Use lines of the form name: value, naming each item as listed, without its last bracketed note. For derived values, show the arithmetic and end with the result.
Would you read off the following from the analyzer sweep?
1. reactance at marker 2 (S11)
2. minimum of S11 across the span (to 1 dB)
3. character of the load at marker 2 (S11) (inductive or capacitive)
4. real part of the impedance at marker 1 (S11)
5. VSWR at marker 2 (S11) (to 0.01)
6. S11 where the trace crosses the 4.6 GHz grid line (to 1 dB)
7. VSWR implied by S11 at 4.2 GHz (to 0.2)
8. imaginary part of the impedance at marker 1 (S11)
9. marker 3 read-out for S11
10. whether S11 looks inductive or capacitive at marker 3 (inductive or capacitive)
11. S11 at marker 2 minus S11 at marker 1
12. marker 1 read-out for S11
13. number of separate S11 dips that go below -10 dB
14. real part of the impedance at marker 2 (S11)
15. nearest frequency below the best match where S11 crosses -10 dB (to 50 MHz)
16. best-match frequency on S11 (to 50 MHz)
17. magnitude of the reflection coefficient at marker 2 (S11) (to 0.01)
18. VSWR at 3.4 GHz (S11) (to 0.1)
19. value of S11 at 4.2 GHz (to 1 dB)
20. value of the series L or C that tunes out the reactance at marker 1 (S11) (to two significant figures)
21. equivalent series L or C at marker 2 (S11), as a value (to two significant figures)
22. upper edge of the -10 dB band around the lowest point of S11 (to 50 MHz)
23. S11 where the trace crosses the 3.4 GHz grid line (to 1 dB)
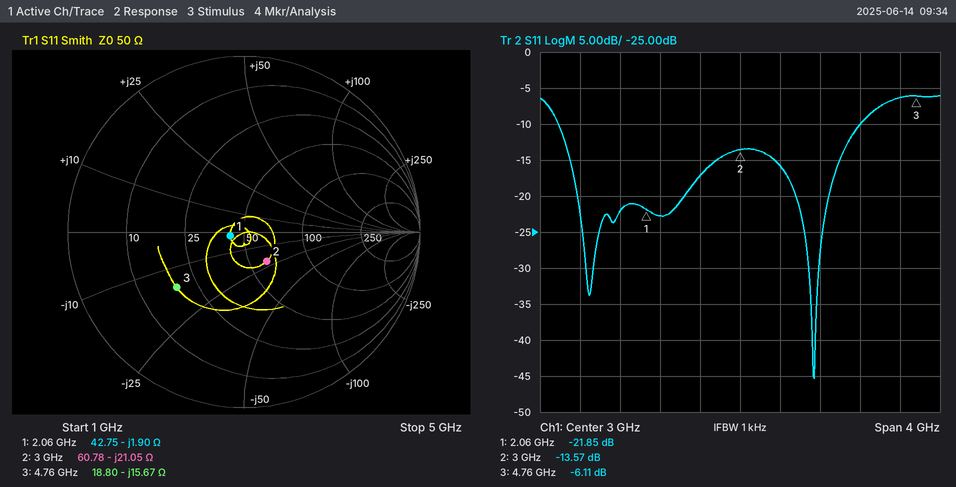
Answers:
reactance at marker 2: -21.05 Ω
minimum of S11 across the span: -45 dB
character of the load at marker 2 (S11): capacitive
real part of the impedance at marker 1: 42.75 Ω
VSWR at marker 2 (S11): (1 + 0.2097)/(1 − 0.2097) ≈ 1.53
S11 where the trace crosses the 4.6 GHz grid line: -6 dB
VSWR implied by S11 at 4.2 GHz: |Γ| = 10^(-10/20) = 0.3162; VSWR = (1 + 0.3162)/(1 − 0.3162) ≈ 1.92, so 2.0 to the nearest 0.2
imaginary part of the impedance at marker 1: -1.90 Ω
marker 3 read-out for S11: -6.11 dB
whether S11 looks inductive or capacitive at marker 3: capacitive
S11 at marker 2 minus S11 at marker 1: -13.57 − (-21.85) = 8.28 dB
marker 1 read-out for S11: -21.85 dB
number of separate S11 dips that go below -10 dB: 2
real part of the impedance at marker 2: 60.78 Ω
nearest frequency below the best match where S11 crosses -10 dB: 1.20 GHz
best-match frequency on S11: 3.75 GHz
magnitude of the reflection coefficient at marker 2 (S11): 0.21
VSWR at 3.4 GHz (S11): |Γ| = 10^(-16/20) = 0.1585; VSWR = (1 + 0.1585)/(1 − 0.1585) ≈ 1.4
value of S11 at 4.2 GHz: -10 dB
value of the series L or C that tunes out the reactance at marker 1 (S11): L = 1.9 Ω/(2π × 2.06 GHz) ≈ 147 pH, so 150 pH to two significant figures
equivalent series L or C at marker 2 (S11), as a value: C = 1/(2π × 3 GHz × 21.05 Ω) ≈ 2.5 pF
upper edge of the -10 dB band around the lowest point of S11: 4.20 GHz
S11 where the trace crosses the 3.4 GHz grid line: -16 dB
